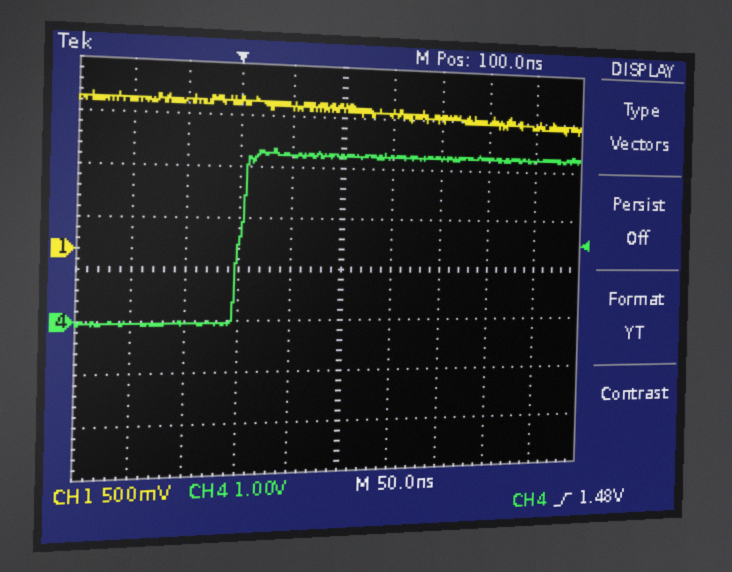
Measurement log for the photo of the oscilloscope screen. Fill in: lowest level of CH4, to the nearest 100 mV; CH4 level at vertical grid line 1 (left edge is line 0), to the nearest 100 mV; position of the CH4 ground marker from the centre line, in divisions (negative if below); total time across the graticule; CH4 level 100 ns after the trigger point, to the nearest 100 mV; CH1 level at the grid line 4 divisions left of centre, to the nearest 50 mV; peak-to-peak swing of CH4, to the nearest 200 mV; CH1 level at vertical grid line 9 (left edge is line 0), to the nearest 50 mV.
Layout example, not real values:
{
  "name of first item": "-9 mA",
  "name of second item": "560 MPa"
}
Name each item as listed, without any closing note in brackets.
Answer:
{
  "lowest level of CH4, to the nearest 100 mV": "-100 mV",
  "CH4 level at vertical grid line 1 (left edge is line 0), to the nearest 100 mV": "0.0 V",
  "position of the CH4 ground marker from the centre line, in divisions": "-1.0 div",
  "total time across the graticule": "500 ns",
  "CH4 level 100 ns after the trigger point, to the nearest 100 mV": "3.2 V",
  "CH1 level at the grid line 4 divisions left of centre, to the nearest 50 mV": "1.40 V",
  "peak-to-peak swing of CH4, to the nearest 200 mV": "3.4 V",
  "CH1 level at vertical grid line 9 (left edge is line 0), to the nearest 50 mV": "1.25 V"
}
